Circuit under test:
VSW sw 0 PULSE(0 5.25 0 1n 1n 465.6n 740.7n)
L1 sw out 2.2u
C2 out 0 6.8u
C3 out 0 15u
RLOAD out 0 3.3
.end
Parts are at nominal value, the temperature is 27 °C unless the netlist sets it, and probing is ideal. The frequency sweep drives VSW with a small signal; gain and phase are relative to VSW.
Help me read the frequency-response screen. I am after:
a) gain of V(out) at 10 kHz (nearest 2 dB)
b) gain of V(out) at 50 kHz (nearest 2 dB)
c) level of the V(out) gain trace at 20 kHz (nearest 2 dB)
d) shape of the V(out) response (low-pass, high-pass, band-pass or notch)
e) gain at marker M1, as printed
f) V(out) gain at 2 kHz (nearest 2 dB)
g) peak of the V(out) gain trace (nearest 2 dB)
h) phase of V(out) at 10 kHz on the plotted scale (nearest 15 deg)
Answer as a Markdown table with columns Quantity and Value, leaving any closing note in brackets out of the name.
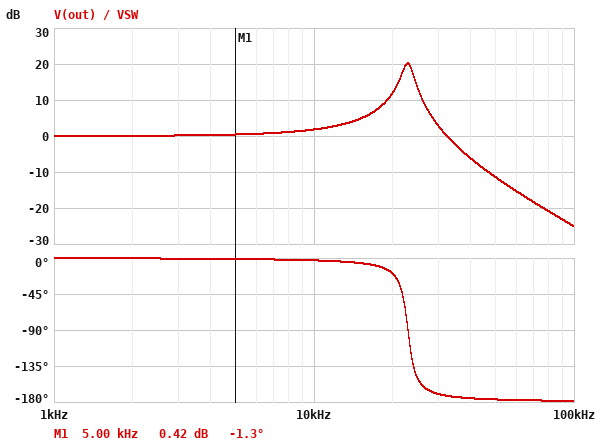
| Quantity | Value |
|---|---|
| gain of V(out) at 10 kHz | 2 dB |
| gain of V(out) at 50 kHz | -12 dB |
| level of the V(out) gain trace at 20 kHz | 12 dB |
| shape of the V(out) response | low-pass |
| gain at marker M1, as printed | 0.42 dB |
| V(out) gain at 2 kHz | 0 dB |
| peak of the V(out) gain trace | 20 dB |
| phase of V(out) at 10 kHz on the plotted scale | 0 deg |
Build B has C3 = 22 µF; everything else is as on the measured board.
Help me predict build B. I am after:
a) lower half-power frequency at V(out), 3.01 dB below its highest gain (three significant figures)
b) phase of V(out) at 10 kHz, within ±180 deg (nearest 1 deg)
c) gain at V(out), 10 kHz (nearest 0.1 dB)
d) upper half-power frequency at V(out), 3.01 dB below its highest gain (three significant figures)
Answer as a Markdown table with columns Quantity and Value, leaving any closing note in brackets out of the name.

| Quantity | Value |
|---|---|
| lower half-power frequency at V(out), 3.01 dB below its highest gain | 19.1 kHz |
| phase of V(out) at 10 kHz, within ±180 deg | -3 deg |
| gain at V(out), 10 kHz | 2.5 dB |
| upper half-power frequency at V(out), 3.01 dB below its highest gain | 20.8 kHz |
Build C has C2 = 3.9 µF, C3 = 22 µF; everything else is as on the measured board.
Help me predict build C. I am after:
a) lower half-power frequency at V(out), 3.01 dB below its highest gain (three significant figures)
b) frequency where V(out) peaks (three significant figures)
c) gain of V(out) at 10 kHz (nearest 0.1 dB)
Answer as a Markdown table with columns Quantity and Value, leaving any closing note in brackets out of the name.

| Quantity | Value |
|---|---|
| lower half-power frequency at V(out), 3.01 dB below its highest gain | 20.1 kHz |
| frequency where V(out) peaks | 21.0 kHz |
| gain of V(out) at 10 kHz | 2.2 dB |
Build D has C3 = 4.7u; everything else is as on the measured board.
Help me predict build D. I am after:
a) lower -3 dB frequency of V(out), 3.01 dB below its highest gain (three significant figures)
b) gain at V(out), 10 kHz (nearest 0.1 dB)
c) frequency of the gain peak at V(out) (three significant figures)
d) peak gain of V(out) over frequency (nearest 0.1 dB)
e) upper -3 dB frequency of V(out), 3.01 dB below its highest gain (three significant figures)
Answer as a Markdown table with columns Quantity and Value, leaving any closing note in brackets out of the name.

| Quantity | Value |
|---|---|
| lower -3 dB frequency of V(out), 3.01 dB below its highest gain | 29.3 kHz |
| gain at V(out), 10 kHz | 0.9 dB |
| frequency of the gain peak at V(out) | 31.5 kHz |
| peak gain of V(out) over frequency | 17.6 dB |
| upper -3 dB frequency of V(out), 3.01 dB below its highest gain | 33.5 kHz |
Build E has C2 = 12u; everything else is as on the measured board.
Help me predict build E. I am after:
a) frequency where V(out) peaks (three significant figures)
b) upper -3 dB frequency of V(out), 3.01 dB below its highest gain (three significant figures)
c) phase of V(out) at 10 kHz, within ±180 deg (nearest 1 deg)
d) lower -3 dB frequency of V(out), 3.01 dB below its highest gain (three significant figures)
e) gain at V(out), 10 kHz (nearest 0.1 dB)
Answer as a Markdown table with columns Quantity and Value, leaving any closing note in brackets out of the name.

| Quantity | Value |
|---|---|
| frequency where V(out) peaks | 20.6 kHz |
| upper -3 dB frequency of V(out), 3.01 dB below its highest gain | 21.5 kHz |
| phase of V(out) at 10 kHz, within ±180 deg | -3 deg |
| lower -3 dB frequency of V(out), 3.01 dB below its highest gain | 19.7 kHz |
| gain at V(out), 10 kHz | 2.3 dB |
